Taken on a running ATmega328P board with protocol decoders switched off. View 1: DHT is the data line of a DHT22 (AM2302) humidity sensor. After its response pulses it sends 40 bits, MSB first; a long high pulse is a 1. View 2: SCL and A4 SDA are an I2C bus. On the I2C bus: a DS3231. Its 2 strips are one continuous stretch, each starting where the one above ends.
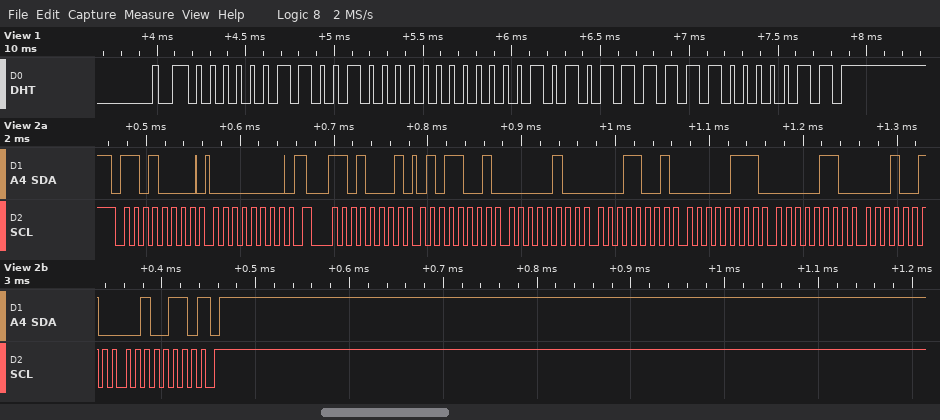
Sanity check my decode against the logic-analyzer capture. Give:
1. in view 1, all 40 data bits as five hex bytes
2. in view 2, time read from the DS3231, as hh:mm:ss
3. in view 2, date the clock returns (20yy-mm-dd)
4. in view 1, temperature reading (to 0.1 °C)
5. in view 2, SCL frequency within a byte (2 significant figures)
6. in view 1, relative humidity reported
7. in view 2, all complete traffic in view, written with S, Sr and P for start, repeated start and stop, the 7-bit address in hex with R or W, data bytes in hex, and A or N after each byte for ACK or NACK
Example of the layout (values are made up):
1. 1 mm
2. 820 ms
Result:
1. 03 20 01 5F 83
2. 19:04:59
3. 2026-12-06
4. 35.1 °C
5. 100 kHz
6. 80.0 %
7. S 68W A 00 A Sr 68R A 59 A 04 A 19 A 07 A 06 A 12 A 26 N P
